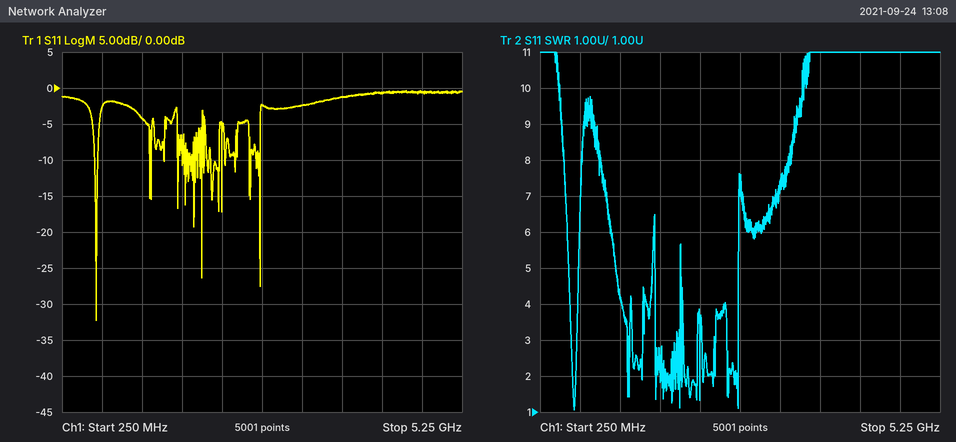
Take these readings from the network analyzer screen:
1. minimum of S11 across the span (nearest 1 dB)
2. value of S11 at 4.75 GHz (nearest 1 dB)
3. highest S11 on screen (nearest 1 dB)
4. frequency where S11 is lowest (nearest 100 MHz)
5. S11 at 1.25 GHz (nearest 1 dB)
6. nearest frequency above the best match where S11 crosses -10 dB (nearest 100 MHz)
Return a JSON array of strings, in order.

["-32 dB", "-1 dB", "0 dB", "700 MHz", "-4 dB", "700 MHz"]
